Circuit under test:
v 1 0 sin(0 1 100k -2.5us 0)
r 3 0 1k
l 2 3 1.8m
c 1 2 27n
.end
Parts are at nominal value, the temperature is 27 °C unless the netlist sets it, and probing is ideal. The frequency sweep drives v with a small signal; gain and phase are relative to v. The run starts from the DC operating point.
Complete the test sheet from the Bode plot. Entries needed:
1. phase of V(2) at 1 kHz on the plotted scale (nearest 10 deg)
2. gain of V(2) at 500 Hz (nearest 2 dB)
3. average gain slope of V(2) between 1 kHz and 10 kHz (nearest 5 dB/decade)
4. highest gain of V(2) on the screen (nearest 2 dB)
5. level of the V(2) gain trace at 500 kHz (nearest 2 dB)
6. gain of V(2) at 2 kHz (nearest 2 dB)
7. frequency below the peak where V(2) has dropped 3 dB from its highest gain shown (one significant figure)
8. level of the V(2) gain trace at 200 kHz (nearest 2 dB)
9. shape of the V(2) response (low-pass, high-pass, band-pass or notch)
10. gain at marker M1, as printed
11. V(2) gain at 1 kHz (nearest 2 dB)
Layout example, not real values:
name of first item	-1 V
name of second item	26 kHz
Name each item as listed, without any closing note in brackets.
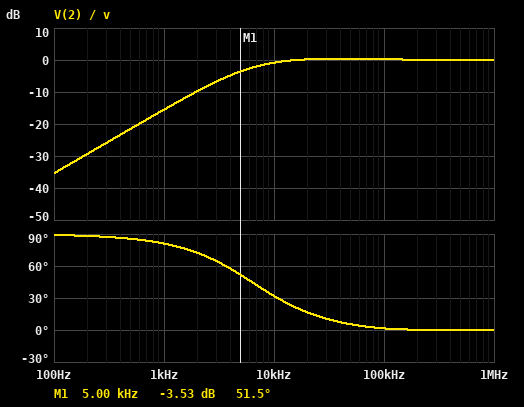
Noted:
phase of V(2) at 1 kHz on the plotted scale	80 deg
gain of V(2) at 500 Hz	-22 dB
average gain slope of V(2) between 1 kHz and 10 kHz	15 dB/decade
highest gain of V(2) on the screen	0 dB
level of the V(2) gain trace at 500 kHz	0 dB
gain of V(2) at 2 kHz	-10 dB
frequency below the peak where V(2) has dropped 3 dB from its highest gain shown	6 kHz
level of the V(2) gain trace at 200 kHz	0 dB
shape of the V(2) response	high-pass
gain at marker M1, as printed	-3.53 dB
V(2) gain at 1 kHz	-16 dB
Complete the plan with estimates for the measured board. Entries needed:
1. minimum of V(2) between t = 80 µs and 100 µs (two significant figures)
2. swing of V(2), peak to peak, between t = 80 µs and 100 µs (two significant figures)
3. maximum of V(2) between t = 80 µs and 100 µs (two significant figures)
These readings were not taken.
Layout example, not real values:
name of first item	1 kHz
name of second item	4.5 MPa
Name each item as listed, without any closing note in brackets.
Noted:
minimum of V(2) between t = 80 µs and 100 µs	-1.1 V
swing of V(2), peak to peak, between t = 80 µs and 100 µs	2.1 V
maximum of V(2) between t = 80 µs and 100 µs	1.0 V
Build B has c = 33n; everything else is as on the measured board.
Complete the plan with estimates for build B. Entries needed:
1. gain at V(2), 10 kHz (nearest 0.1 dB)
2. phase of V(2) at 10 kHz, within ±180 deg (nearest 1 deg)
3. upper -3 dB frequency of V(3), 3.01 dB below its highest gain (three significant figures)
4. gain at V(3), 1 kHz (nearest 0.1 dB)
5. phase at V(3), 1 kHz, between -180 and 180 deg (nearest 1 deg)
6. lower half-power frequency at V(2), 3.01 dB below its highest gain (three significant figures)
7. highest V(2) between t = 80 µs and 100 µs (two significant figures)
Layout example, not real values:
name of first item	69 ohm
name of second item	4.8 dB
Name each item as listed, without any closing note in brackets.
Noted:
gain at V(2), 10 kHz	-0.5 dB
phase of V(2) at 10 kHz, within ±180 deg	27 deg
upper -3 dB frequency of V(3), 3.01 dB below its highest gain	93.0 kHz
gain at V(3), 1 kHz	-13.8 dB
phase at V(3), 1 kHz, between -180 and 180 deg	78 deg
lower half-power frequency at V(2), 3.01 dB below its highest gain	4.94 kHz
highest V(2) between t = 80 µs and 100 µs	980 mV
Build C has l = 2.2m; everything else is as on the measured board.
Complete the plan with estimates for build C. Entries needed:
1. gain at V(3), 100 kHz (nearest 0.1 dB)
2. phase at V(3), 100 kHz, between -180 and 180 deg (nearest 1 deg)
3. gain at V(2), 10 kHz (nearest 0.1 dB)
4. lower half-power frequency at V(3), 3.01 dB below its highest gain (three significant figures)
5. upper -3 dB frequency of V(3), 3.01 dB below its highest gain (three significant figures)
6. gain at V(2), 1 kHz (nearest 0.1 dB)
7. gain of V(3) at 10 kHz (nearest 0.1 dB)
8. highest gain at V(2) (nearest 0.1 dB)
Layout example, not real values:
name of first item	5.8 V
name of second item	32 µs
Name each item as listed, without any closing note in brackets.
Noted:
gain at V(3), 100 kHz	-4.4 dB
phase at V(3), 100 kHz, between -180 and 180 deg	-53 deg
gain at V(2), 10 kHz	-0.7 dB
lower half-power frequency at V(3), 3.01 dB below its highest gain	5.48 kHz
upper -3 dB frequency of V(3), 3.01 dB below its highest gain	77.8 kHz
gain at V(2), 1 kHz	-15.5 dB
gain of V(3) at 10 kHz	-0.8 dB
highest gain at V(2)	0.5 dB
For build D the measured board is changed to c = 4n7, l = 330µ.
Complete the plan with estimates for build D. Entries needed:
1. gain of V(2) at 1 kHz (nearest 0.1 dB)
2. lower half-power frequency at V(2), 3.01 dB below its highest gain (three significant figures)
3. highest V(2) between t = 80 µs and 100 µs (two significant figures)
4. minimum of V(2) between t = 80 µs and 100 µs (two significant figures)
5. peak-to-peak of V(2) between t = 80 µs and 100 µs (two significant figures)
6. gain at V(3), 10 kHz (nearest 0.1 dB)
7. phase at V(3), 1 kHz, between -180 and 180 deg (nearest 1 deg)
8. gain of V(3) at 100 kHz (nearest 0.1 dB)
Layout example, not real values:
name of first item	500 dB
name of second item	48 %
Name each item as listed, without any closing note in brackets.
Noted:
gain of V(2) at 1 kHz	-30.6 dB
lower half-power frequency at V(2), 3.01 dB below its highest gain	34.7 kHz
highest V(2) between t = 80 µs and 100 µs	1.0 V
minimum of V(2) between t = 80 µs and 100 µs	-1.0 V
peak-to-peak of V(2) between t = 80 µs and 100 µs	2.0 V
gain at V(3), 10 kHz	-10.9 dB
phase at V(3), 1 kHz, between -180 and 180 deg	88 deg
gain of V(3) at 100 kHz	-0.1 dB
